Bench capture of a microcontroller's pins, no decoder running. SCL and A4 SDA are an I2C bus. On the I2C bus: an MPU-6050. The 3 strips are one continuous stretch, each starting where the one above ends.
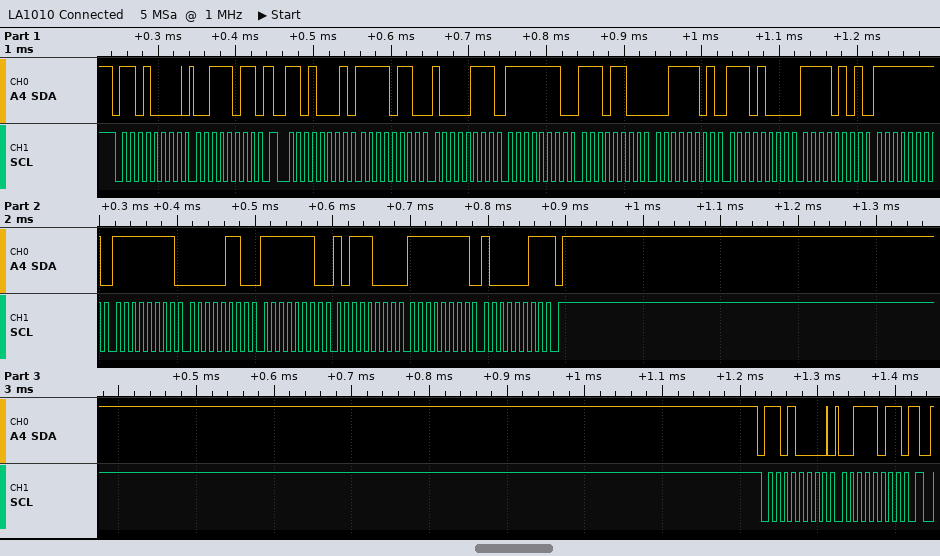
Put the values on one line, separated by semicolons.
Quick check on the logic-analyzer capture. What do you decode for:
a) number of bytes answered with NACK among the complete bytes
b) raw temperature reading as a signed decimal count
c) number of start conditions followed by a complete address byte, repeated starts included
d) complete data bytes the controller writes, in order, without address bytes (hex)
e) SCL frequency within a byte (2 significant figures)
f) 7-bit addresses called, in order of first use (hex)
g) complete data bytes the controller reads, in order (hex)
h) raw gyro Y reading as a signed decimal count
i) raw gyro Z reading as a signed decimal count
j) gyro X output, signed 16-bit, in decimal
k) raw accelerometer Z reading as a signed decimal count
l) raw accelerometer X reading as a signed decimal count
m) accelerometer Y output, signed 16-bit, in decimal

1; -2561; 3; 3B 3B; 100 kHz; 0x68; F6 87 FE EC 3D E8 F5 FF FF 06 FE B8 FF 83; -328; -125; -250; 15848; -2425; -276
